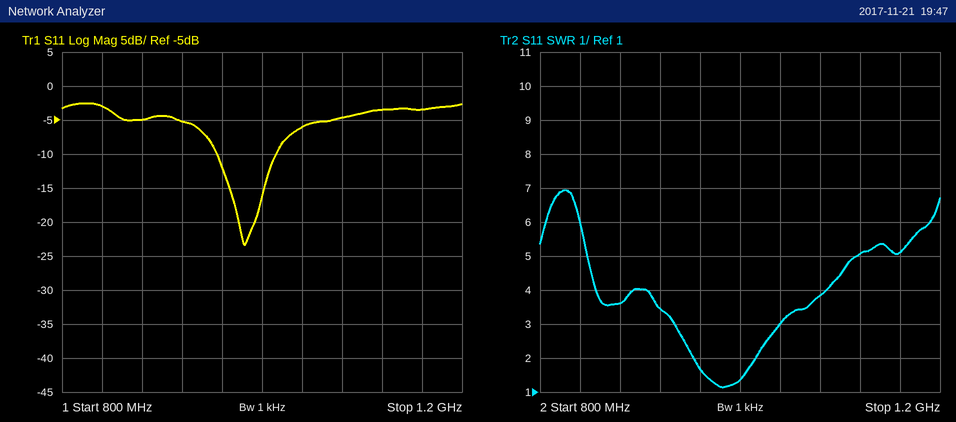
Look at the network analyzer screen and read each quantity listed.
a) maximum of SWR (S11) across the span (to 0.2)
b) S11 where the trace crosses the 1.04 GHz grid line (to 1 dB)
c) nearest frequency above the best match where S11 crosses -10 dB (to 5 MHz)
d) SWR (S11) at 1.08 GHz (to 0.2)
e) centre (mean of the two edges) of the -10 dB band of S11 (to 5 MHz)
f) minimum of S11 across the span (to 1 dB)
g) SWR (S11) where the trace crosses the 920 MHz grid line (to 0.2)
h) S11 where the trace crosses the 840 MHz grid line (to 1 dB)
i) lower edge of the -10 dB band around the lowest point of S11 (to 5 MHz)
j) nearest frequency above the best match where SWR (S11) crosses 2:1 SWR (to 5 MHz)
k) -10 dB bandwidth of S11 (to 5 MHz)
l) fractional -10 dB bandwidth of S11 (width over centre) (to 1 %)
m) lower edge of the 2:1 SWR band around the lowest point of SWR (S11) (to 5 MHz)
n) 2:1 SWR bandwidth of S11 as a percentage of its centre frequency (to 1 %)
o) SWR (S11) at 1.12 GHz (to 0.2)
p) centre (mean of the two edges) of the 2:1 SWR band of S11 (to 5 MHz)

7.0
-6 dB
1.015 GHz
3.8
985 MHz
-23 dB
3.4
-3 dB
955 MHz
1.015 GHz
60 MHz
6 %
955 MHz
6 %
5.0
985 MHz
